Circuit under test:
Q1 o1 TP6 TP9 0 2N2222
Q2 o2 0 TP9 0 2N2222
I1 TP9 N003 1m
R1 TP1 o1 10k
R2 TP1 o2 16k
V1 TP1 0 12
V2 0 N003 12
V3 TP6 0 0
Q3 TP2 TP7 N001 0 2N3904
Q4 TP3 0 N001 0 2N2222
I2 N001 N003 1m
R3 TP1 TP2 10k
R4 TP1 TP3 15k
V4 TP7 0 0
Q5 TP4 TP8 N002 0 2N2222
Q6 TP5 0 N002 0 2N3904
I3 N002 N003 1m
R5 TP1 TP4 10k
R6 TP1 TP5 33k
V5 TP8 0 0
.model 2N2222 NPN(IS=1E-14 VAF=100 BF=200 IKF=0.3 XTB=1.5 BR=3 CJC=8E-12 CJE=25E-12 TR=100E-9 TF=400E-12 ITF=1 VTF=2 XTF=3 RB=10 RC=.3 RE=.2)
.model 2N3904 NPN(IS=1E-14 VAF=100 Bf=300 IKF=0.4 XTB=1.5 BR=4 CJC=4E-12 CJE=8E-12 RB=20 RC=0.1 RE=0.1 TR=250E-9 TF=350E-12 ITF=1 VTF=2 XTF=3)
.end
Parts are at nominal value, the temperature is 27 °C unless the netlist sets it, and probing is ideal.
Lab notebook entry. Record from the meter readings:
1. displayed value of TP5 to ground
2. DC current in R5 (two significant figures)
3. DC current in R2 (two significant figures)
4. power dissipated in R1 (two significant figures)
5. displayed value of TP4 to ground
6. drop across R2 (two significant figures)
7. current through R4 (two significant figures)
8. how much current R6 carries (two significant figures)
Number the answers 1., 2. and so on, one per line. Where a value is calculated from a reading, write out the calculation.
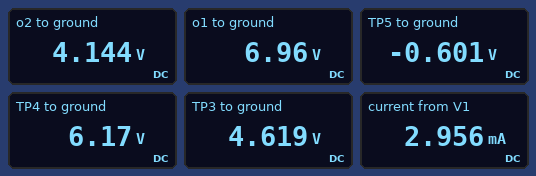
1. -0.601 V
2. (12 V - 6.17 V) / 10 kΩ = 580 µA
3. (12 V - 4.144 V) / 16 kΩ = 490 µA
4. (12 V - 6.96 V)^2 / 10 kΩ = 2.5 mW
5. 6.17 V
6. 12 V - 4.144 V = 7.9 V
7. (12 V - 4.619 V) / 15 kΩ = 490 µA
8. (12 V - (-601 mV)) / 33 kΩ = 380 µA
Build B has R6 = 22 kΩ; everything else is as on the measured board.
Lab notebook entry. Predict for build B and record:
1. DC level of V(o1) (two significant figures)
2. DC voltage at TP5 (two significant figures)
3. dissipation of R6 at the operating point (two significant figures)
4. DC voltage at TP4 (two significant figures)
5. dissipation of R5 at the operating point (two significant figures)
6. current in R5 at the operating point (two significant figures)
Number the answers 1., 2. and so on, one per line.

1. 7.0 V
2. 1.3 V
3. 5.2 mW
4. 6.9 V
5. 2.6 mW
6. 510 µA
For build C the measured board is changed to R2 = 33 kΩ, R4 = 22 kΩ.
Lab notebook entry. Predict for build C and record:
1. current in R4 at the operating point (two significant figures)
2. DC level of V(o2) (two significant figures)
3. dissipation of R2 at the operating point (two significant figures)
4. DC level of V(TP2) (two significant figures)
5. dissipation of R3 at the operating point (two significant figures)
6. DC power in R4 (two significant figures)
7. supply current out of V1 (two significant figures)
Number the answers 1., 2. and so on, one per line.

1. 480 µA
2. -600 mV
3. 4.8 mW
4. 6.9 V
5. 2.6 mW
6. 5.2 mW
7. 2.9 mA
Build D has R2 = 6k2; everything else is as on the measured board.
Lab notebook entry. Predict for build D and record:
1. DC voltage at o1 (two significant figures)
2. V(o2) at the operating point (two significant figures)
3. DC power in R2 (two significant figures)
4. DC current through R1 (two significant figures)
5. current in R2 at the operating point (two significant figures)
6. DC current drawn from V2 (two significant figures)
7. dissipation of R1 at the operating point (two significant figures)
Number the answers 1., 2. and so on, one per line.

1. 7.1 V
2. 8.9 V
3. 1.6 mW
4. 490 µA
5. 500 µA
6. 3.0 mA
7. 2.4 mW
